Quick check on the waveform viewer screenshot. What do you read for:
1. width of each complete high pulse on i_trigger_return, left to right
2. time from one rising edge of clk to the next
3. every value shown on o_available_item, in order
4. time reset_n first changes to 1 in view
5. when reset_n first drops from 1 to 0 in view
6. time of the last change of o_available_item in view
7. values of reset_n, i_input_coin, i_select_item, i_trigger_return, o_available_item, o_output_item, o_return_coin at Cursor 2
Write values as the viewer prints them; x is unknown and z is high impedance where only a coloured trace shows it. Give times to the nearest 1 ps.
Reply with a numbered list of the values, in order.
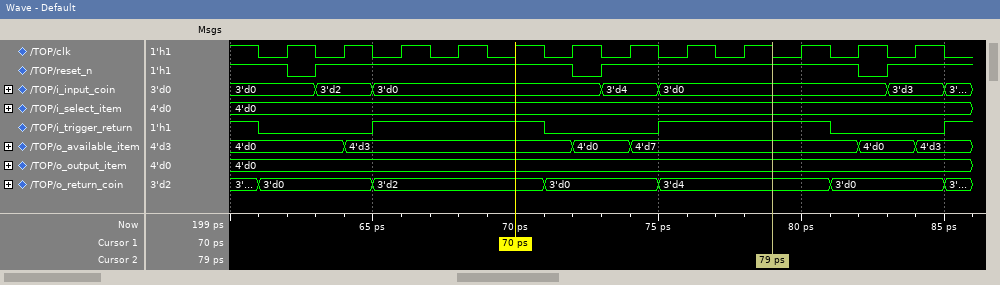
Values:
1. 6 ps, 6 ps
2. 2 ps
3. 4'd0, 4'd3, 4'd0, 4'd7, 4'd0, 4'd3
4. 63 ps
5. 62 ps
6. 84 ps
7. reset_n=1, i_input_coin=3'd0, i_select_item=4'd0, i_trigger_return=1, o_available_item=4'd7, o_output_item=4'd0, o_return_coin=3'd4
